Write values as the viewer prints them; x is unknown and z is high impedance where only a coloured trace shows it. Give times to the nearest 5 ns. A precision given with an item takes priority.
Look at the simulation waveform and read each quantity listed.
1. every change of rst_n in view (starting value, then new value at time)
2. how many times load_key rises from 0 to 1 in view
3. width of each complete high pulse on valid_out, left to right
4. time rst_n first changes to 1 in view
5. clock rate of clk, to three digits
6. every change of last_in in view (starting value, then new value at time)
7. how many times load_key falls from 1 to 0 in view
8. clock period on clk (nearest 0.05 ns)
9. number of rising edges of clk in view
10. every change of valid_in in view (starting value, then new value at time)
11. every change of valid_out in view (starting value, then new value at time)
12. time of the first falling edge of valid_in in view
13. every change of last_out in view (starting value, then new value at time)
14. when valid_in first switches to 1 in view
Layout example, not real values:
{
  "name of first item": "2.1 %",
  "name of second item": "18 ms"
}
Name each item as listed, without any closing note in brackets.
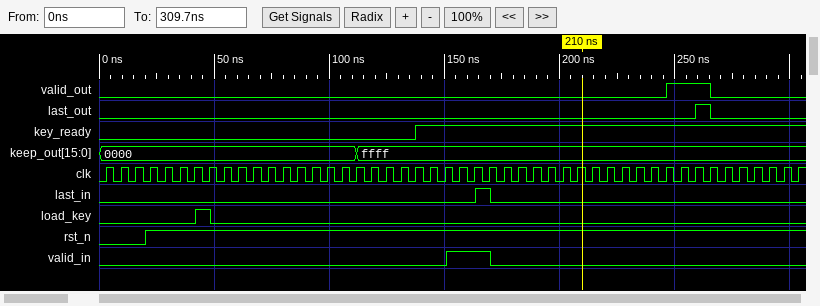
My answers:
{
  "every change of rst_n in view": "0, 1 at 20 ns",
  "how many times load_key rises from 0 to 1 in view": "1",
  "width of each complete high pulse on valid_out, left to right": "20 ns",
  "time rst_n first changes to 1 in view": "20 ns",
  "clock rate of clk, to three digits": "156 MHz",
  "every change of last_in in view": "0, 1 at 165 ns, 0 at 170 ns",
  "how many times load_key falls from 1 to 0 in view": "1",
  "clock period on clk": "6.4 ns",
  "number of rising edges of clk in view": "48",
  "every change of valid_in in view": "0, 1 at 150 ns, 0 at 170 ns",
  "every change of valid_out in view": "0, 1 at 245 ns, 0 at 265 ns",
  "time of the first falling edge of valid_in in view": "170 ns",
  "every change of last_out in view": "0, 1 at 260 ns, 0 at 265 ns",
  "when valid_in first switches to 1 in view": "150 ns"
}
